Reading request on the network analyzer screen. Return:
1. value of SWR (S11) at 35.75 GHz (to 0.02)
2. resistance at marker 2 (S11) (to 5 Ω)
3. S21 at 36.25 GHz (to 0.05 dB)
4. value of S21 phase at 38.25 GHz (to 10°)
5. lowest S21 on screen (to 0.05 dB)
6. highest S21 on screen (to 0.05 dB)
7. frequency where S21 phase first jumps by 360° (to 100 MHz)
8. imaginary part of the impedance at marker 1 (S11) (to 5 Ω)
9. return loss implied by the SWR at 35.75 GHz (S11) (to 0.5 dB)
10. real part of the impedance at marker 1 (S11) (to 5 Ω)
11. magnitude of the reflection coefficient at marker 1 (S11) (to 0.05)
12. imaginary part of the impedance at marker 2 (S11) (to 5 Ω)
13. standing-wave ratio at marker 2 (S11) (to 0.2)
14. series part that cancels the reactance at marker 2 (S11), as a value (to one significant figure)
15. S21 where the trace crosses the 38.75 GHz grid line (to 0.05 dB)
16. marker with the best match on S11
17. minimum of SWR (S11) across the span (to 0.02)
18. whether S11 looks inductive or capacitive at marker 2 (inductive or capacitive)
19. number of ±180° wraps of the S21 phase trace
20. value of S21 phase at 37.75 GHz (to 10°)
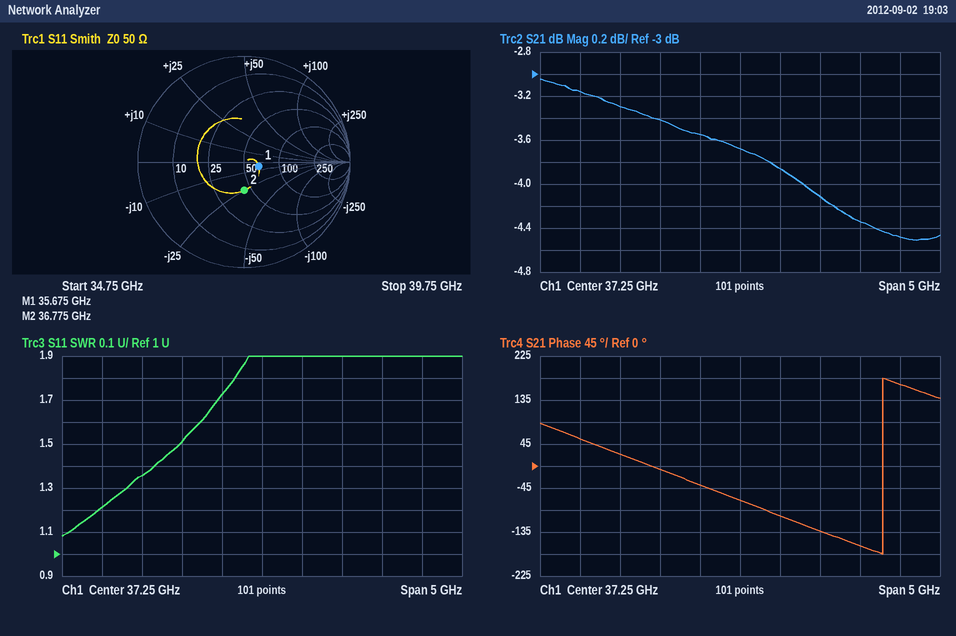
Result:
1.36
45 Ω
-3.40 dB
-130°
-4.50 dB
-3.05 dB
39.0 GHz
-5 Ω
16.5 dB
65 Ω
0.15
-25 Ω
1.8
100 pH
-4.35 dB
marker 1
1.08
capacitive
1
-100°
